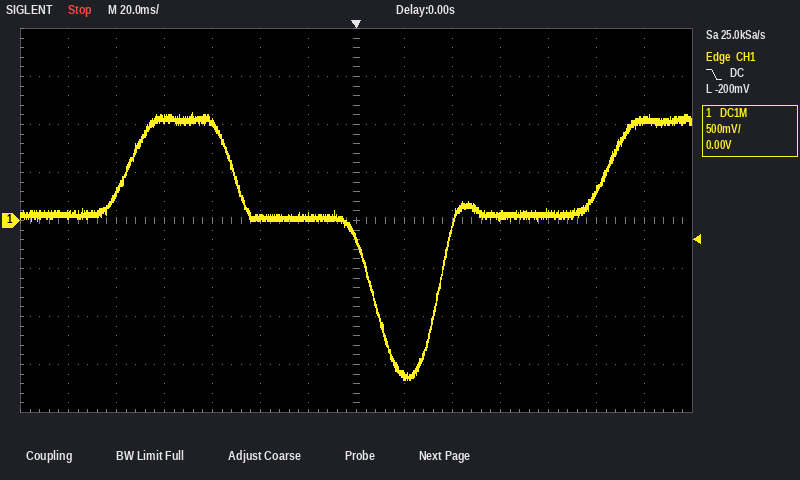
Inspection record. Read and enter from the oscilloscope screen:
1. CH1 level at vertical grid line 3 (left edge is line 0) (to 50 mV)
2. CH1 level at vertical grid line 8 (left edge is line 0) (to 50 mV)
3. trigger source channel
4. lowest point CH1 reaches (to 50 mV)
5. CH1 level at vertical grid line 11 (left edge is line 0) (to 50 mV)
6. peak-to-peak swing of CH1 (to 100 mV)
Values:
1.05 V
-1.60 V
CH1
-1.65 V
50 mV
2.80 V
